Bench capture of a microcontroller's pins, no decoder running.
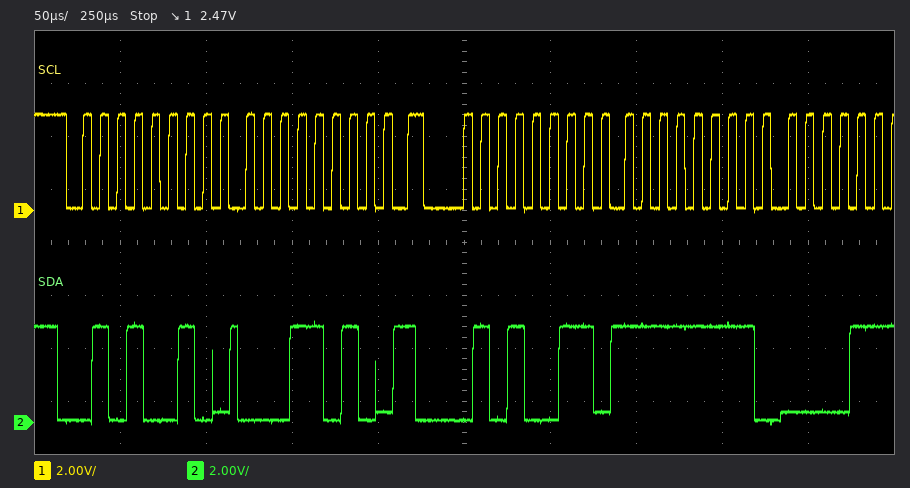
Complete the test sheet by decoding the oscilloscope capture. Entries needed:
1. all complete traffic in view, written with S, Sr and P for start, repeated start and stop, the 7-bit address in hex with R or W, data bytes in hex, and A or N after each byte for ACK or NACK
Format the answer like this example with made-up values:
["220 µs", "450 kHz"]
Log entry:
["S 29W A 1A A Sr 29R A FF A"]
